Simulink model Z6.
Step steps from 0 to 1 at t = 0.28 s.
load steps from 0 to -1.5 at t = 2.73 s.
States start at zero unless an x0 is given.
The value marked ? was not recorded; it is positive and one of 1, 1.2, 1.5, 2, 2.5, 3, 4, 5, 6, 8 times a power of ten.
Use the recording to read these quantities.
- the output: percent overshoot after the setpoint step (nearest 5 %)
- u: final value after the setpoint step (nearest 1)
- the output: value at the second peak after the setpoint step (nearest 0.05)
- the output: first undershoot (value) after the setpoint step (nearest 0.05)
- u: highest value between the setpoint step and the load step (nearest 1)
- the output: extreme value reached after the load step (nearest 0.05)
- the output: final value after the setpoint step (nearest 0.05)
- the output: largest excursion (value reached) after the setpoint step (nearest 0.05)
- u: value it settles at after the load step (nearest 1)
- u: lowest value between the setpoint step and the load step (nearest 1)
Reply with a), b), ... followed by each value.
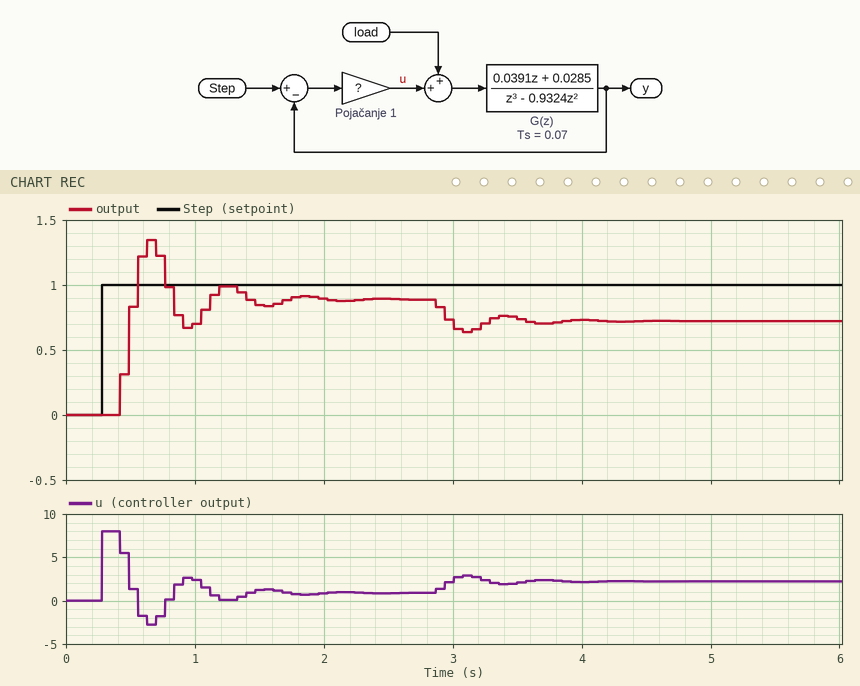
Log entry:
a) 50 %
b) 1
c) 1.00
d) 0.65
e) 8
f) 0.65
g) 0.90
h) 1.35
i) 2
j) -3
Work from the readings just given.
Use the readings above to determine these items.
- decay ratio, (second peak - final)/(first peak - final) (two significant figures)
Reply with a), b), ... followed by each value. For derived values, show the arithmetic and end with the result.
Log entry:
a) (1 - 0.9) / (1.35 - 0.9) = 0.22
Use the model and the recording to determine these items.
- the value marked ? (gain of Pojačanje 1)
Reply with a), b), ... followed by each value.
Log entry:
a) 8
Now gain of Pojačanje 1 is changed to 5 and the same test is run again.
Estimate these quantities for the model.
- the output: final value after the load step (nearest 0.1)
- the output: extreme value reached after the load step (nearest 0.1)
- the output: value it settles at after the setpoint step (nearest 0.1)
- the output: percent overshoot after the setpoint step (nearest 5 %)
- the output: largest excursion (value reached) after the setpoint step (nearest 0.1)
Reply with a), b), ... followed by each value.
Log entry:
a) 0.6
b) 0.5
c) 0.8
d) 20 %
e) 1.0
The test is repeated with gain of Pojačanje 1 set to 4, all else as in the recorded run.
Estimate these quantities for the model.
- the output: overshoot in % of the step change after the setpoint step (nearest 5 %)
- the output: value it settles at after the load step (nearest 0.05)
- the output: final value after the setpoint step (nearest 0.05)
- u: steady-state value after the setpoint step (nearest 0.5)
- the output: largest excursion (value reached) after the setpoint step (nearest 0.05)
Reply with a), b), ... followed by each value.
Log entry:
a) 10 %
b) 0.50
c) 0.80
d) 1.0
e) 0.85
